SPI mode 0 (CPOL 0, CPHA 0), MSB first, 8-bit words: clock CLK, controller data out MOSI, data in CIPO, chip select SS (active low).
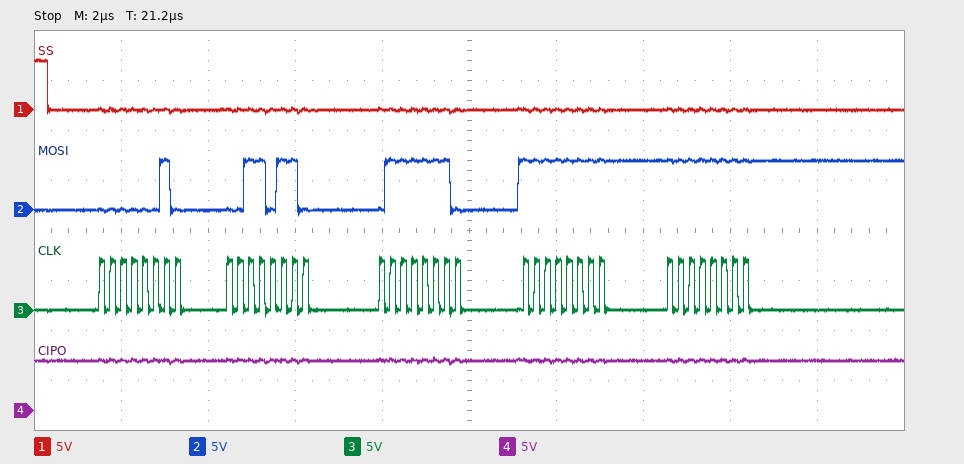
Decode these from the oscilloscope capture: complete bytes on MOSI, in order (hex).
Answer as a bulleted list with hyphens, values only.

- 0x02 0x36 0x7E 0xFF 0xFF
